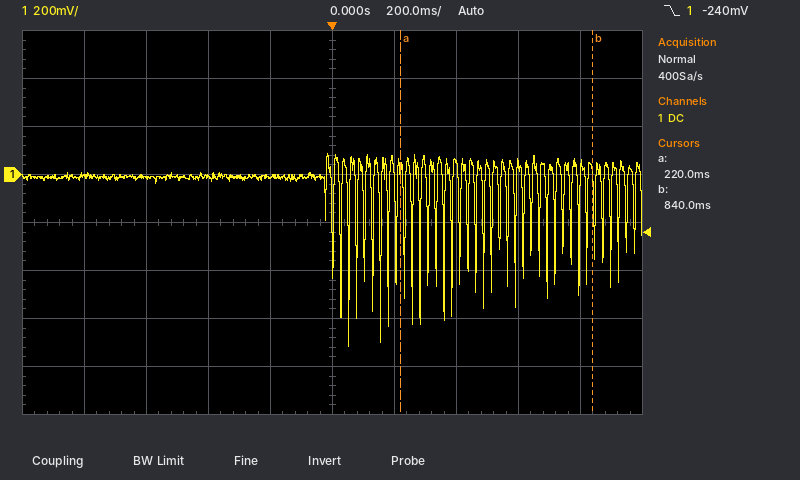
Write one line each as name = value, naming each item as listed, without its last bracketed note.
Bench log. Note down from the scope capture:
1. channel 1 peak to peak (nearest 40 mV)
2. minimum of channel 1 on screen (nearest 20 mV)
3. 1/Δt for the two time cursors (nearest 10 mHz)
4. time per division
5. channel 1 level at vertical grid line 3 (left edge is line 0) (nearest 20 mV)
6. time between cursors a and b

channel 1 peak to peak = 800 mV
minimum of channel 1 on screen = -720 mV
1/Δt for the two time cursors = 1.61 Hz
time per division = 200 ms
channel 1 level at vertical grid line 3 (left edge is line 0) = 0 mV
time between cursors a and b = 620 ms
